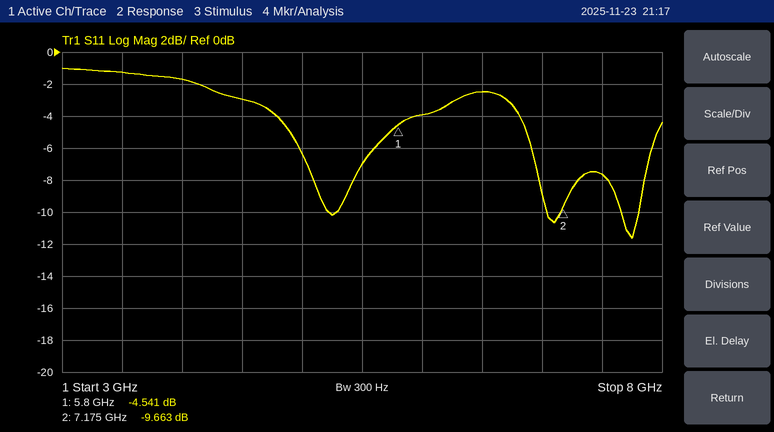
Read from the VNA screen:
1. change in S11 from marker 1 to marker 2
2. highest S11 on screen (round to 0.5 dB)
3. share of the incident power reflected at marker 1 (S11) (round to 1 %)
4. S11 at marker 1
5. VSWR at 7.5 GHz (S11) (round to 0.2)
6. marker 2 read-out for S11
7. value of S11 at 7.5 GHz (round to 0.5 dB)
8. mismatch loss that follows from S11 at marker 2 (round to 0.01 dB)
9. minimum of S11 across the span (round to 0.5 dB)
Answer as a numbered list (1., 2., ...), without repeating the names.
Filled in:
1. -5.122 dB
2. -1.0 dB
3. 35 %
4. -4.541 dB
5. 2.4
6. -9.663 dB
7. -7.5 dB
8. 0.50 dB
9. -11.5 dB
